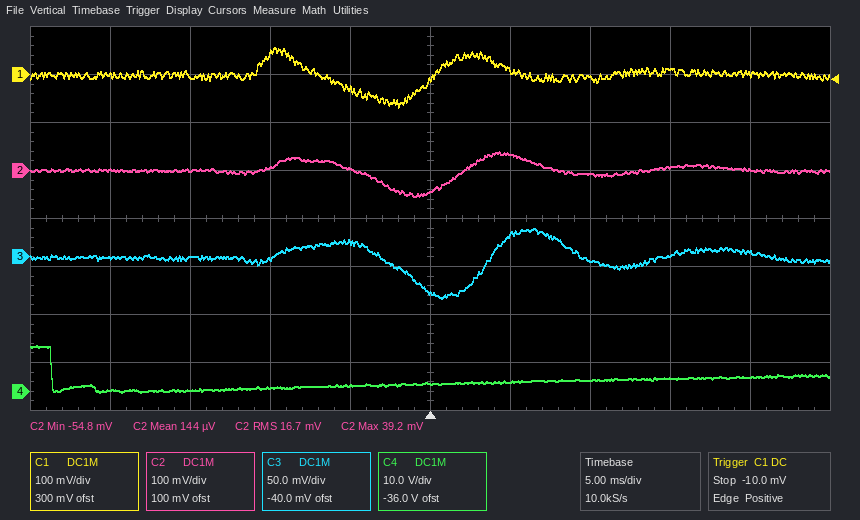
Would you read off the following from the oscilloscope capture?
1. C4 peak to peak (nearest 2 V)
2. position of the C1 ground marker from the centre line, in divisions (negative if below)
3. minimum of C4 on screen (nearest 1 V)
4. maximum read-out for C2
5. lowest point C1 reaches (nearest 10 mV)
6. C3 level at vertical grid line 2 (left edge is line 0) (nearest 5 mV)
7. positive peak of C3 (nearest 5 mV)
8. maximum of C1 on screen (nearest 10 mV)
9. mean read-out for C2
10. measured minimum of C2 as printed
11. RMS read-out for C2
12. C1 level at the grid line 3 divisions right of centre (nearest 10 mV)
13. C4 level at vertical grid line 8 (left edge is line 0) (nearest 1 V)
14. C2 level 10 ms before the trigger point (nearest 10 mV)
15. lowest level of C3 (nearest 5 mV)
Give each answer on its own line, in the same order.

10 V
+3.0 div
0 V
39.2 mV
-70 mV
0 mV
30 mV
60 mV
144 µV
-54.8 mV
16.7 mV
10 mV
3 V
10 mV
-45 mV
